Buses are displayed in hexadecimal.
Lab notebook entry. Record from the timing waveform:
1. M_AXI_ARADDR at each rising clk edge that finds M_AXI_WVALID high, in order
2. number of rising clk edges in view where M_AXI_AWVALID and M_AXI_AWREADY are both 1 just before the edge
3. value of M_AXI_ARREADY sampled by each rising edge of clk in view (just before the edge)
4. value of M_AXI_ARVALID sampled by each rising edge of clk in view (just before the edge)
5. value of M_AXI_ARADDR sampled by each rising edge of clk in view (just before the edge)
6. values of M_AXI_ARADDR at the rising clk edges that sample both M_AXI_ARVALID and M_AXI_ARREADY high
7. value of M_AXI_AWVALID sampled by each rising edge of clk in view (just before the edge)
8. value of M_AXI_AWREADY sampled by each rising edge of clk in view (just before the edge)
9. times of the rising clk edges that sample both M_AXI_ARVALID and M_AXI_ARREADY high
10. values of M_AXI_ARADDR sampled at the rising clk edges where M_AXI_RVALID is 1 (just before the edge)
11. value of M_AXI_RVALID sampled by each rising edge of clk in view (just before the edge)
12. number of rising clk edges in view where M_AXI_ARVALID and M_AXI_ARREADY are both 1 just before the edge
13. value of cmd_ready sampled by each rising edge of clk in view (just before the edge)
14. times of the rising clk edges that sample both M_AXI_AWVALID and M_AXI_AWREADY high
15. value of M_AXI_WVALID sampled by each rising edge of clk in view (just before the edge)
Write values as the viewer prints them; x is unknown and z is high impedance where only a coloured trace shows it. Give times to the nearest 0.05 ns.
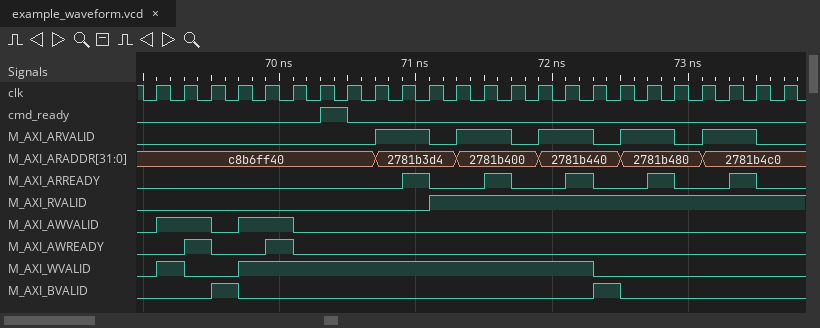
c8b6ff40, c8b6ff40, c8b6ff40, c8b6ff40, c8b6ff40, c8b6ff40, 2781b3d4, 2781b3d4, 2781b3d4, 2781b400, 2781b400, 2781b400, 2781b440, 2781b440
2
0 0 0 0 0 0 0 0 0 0 1 0 0 1 0 0 1 0 0 1 0 0 1 0
0 0 0 0 0 0 0 0 0 1 1 0 1 1 0 1 1 0 1 1 0 1 1 0
c8b6ff40, c8b6ff40, c8b6ff40, c8b6ff40, c8b6ff40, c8b6ff40, c8b6ff40, c8b6ff40, c8b6ff40, 2781b3d4, 2781b3d4, 2781b3d4, 2781b400, 2781b400, 2781b400, 2781b440, 2781b440, 2781b440, 2781b480, 2781b480, 2781b480, 2781b4c0, 2781b4c0, 2781b4c0
2781b3d4, 2781b400, 2781b440, 2781b480, 2781b4c0
0 1 1 0 1 1 0 0 0 0 0 0 0 0 0 0 0 0 0 0 0 0 0 0
0 0 1 0 0 1 0 0 0 0 0 0 0 0 0 0 0 0 0 0 0 0 0 0
71.1 ns, 71.7 ns, 72.3 ns, 72.9 ns, 73.5 ns
2781b3d4, 2781b400, 2781b400, 2781b400, 2781b440, 2781b440, 2781b440, 2781b480, 2781b480, 2781b480, 2781b4c0, 2781b4c0, 2781b4c0
0 0 0 0 0 0 0 0 0 0 0 1 1 1 1 1 1 1 1 1 1 1 1 1
5
0 0 0 0 0 0 0 1 0 0 0 0 0 0 0 0 0 0 0 0 0 0 0 0
69.5 ns, 70.1 ns
0 1 0 0 1 1 1 1 1 1 1 1 1 1 1 1 1 0 0 0 0 0 0 0
